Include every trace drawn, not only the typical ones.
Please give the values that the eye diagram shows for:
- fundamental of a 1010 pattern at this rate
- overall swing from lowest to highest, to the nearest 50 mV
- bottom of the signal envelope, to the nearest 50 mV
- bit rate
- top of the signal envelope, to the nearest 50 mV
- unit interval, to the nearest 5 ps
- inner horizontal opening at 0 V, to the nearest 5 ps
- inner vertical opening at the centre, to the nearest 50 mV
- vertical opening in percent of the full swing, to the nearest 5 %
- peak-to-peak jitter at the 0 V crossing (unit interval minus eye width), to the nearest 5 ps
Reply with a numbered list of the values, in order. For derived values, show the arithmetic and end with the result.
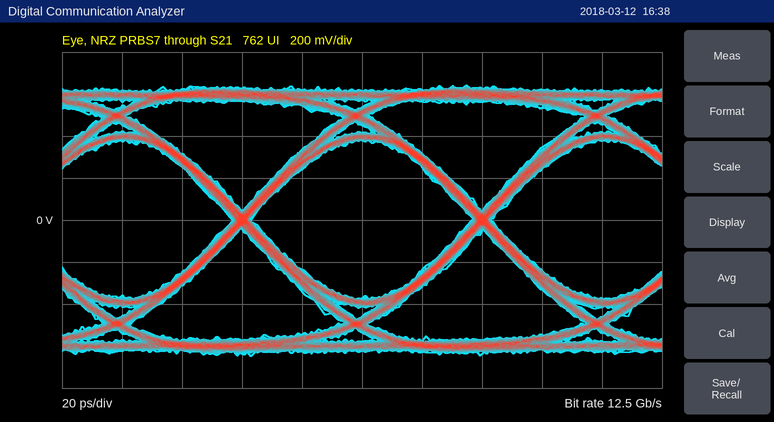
1. 6.25 GHz
2. 1.30 V
3. -650 mV
4. 12.5 Gb/s
5. 650 mV
6. 80 ps
7. 75 ps
8. 750 mV
9. 750 mV / 1.30 V ≈ 57.7 %, so 60 % to the nearest 5 %
10. 5 ps
